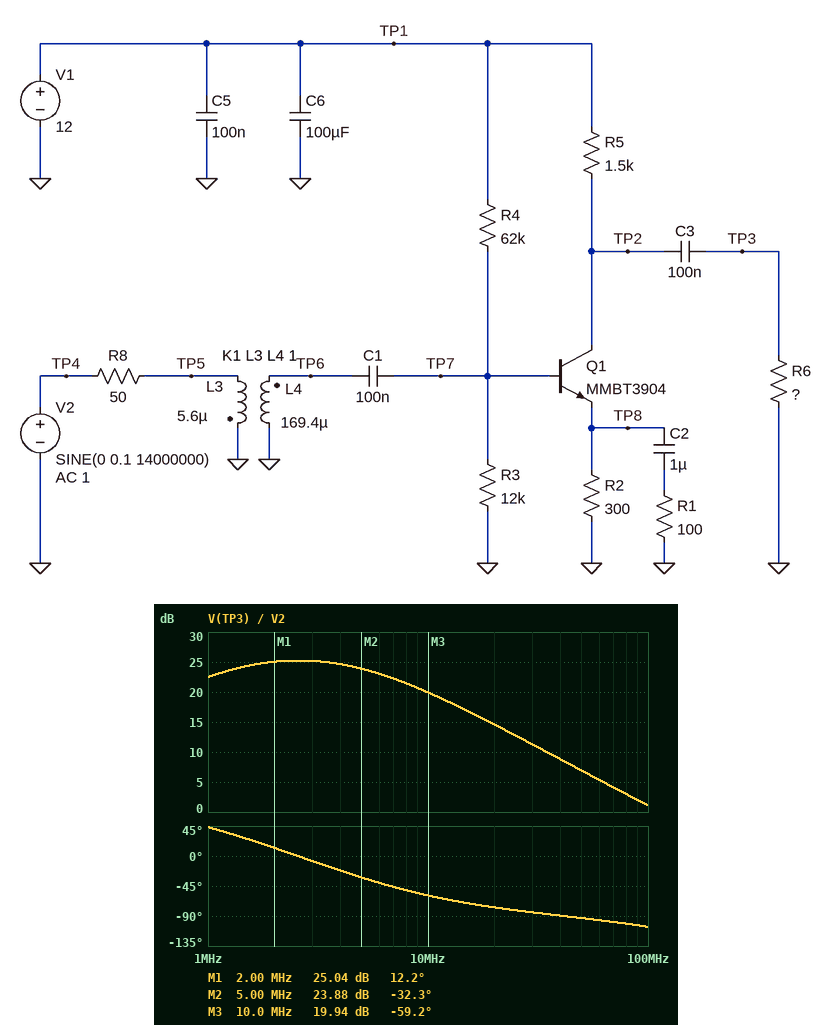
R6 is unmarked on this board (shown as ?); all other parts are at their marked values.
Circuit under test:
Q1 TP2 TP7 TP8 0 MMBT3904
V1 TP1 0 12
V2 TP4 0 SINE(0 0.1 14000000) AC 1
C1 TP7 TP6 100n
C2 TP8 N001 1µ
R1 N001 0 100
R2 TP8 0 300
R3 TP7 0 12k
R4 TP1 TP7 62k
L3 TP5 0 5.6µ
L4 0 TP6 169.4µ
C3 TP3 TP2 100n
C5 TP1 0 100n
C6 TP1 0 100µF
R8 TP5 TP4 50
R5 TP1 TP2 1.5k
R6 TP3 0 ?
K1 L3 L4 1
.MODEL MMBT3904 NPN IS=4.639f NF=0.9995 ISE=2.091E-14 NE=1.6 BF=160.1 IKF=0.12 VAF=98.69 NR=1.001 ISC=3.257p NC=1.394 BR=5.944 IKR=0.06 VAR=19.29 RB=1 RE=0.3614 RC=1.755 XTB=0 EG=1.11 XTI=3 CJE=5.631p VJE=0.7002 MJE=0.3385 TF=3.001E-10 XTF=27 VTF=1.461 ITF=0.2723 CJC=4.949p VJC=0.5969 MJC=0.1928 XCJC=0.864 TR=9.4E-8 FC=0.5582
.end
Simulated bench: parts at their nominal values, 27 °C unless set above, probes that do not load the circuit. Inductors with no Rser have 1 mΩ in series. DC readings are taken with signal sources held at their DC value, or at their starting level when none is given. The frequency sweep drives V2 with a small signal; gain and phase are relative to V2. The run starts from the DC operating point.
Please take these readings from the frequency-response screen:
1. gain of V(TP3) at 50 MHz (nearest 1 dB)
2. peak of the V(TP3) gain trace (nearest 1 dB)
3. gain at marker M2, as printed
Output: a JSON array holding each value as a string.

["7 dB", "25 dB", "23.88 dB"]
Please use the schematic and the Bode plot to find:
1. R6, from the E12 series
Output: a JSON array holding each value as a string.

["470 Ω"]
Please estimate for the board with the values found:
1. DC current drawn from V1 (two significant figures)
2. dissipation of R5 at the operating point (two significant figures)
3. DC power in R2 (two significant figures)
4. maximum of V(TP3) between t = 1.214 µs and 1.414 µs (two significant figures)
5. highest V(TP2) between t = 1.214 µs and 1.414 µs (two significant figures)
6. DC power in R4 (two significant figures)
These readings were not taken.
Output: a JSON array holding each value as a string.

["3.5 mA", "17 mW", "3.5 mW", "720 mV", "7.7 V", "1.7 mW"]
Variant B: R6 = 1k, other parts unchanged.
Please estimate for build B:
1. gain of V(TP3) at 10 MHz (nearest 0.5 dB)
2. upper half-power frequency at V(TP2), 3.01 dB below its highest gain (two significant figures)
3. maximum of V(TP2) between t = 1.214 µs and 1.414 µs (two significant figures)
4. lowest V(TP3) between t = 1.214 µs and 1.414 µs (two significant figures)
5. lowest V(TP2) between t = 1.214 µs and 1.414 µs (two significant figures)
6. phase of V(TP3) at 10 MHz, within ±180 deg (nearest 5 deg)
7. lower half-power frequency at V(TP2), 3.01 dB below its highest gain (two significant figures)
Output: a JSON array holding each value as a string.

["22.0 dB", "5.1 MHz", "7.8 V", "-900 mV", "6.0 V", "-70 deg", "910 kHz"]
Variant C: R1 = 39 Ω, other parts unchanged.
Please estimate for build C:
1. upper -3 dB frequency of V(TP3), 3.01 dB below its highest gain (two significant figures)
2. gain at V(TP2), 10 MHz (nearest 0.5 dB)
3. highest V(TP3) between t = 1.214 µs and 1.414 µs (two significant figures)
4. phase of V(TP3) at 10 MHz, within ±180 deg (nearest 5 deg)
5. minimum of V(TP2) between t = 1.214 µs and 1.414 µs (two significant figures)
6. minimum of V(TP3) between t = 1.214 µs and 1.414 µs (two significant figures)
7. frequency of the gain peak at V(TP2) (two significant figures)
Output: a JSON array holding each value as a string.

["4.5 MHz", "21.5 dB", "800 mV", "-70 deg", "6.1 V", "-880 mV", "1.9 MHz"]
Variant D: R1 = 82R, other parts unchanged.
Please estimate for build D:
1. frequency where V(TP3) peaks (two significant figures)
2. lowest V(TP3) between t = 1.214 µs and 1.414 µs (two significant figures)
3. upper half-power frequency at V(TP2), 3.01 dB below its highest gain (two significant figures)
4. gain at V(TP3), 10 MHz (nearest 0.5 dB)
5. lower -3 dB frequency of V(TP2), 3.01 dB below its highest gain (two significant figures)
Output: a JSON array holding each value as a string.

["2.4 MHz", "-780 mV", "6.4 MHz", "20.5 dB", "930 kHz"]
